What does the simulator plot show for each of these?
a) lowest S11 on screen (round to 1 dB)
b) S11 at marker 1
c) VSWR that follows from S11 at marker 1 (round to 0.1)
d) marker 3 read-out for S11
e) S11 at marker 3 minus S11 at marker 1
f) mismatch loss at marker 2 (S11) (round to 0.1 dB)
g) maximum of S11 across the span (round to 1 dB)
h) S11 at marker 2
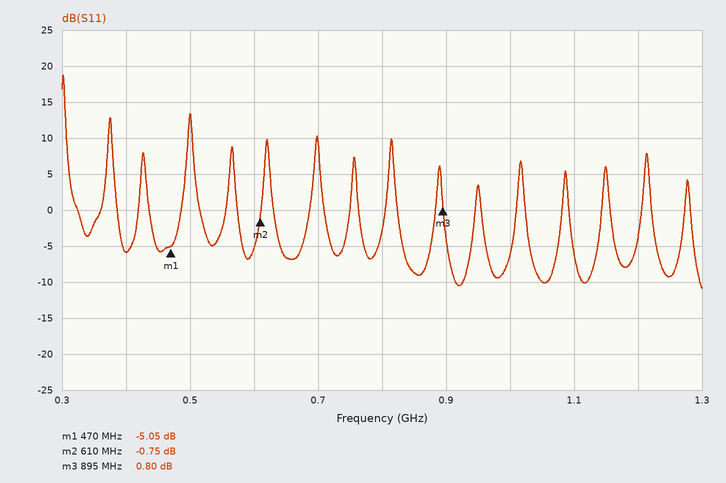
-11 dB
-5.05 dB
3.5
0.80 dB
5.85 dB
8.0 dB
19 dB
-0.75 dB
